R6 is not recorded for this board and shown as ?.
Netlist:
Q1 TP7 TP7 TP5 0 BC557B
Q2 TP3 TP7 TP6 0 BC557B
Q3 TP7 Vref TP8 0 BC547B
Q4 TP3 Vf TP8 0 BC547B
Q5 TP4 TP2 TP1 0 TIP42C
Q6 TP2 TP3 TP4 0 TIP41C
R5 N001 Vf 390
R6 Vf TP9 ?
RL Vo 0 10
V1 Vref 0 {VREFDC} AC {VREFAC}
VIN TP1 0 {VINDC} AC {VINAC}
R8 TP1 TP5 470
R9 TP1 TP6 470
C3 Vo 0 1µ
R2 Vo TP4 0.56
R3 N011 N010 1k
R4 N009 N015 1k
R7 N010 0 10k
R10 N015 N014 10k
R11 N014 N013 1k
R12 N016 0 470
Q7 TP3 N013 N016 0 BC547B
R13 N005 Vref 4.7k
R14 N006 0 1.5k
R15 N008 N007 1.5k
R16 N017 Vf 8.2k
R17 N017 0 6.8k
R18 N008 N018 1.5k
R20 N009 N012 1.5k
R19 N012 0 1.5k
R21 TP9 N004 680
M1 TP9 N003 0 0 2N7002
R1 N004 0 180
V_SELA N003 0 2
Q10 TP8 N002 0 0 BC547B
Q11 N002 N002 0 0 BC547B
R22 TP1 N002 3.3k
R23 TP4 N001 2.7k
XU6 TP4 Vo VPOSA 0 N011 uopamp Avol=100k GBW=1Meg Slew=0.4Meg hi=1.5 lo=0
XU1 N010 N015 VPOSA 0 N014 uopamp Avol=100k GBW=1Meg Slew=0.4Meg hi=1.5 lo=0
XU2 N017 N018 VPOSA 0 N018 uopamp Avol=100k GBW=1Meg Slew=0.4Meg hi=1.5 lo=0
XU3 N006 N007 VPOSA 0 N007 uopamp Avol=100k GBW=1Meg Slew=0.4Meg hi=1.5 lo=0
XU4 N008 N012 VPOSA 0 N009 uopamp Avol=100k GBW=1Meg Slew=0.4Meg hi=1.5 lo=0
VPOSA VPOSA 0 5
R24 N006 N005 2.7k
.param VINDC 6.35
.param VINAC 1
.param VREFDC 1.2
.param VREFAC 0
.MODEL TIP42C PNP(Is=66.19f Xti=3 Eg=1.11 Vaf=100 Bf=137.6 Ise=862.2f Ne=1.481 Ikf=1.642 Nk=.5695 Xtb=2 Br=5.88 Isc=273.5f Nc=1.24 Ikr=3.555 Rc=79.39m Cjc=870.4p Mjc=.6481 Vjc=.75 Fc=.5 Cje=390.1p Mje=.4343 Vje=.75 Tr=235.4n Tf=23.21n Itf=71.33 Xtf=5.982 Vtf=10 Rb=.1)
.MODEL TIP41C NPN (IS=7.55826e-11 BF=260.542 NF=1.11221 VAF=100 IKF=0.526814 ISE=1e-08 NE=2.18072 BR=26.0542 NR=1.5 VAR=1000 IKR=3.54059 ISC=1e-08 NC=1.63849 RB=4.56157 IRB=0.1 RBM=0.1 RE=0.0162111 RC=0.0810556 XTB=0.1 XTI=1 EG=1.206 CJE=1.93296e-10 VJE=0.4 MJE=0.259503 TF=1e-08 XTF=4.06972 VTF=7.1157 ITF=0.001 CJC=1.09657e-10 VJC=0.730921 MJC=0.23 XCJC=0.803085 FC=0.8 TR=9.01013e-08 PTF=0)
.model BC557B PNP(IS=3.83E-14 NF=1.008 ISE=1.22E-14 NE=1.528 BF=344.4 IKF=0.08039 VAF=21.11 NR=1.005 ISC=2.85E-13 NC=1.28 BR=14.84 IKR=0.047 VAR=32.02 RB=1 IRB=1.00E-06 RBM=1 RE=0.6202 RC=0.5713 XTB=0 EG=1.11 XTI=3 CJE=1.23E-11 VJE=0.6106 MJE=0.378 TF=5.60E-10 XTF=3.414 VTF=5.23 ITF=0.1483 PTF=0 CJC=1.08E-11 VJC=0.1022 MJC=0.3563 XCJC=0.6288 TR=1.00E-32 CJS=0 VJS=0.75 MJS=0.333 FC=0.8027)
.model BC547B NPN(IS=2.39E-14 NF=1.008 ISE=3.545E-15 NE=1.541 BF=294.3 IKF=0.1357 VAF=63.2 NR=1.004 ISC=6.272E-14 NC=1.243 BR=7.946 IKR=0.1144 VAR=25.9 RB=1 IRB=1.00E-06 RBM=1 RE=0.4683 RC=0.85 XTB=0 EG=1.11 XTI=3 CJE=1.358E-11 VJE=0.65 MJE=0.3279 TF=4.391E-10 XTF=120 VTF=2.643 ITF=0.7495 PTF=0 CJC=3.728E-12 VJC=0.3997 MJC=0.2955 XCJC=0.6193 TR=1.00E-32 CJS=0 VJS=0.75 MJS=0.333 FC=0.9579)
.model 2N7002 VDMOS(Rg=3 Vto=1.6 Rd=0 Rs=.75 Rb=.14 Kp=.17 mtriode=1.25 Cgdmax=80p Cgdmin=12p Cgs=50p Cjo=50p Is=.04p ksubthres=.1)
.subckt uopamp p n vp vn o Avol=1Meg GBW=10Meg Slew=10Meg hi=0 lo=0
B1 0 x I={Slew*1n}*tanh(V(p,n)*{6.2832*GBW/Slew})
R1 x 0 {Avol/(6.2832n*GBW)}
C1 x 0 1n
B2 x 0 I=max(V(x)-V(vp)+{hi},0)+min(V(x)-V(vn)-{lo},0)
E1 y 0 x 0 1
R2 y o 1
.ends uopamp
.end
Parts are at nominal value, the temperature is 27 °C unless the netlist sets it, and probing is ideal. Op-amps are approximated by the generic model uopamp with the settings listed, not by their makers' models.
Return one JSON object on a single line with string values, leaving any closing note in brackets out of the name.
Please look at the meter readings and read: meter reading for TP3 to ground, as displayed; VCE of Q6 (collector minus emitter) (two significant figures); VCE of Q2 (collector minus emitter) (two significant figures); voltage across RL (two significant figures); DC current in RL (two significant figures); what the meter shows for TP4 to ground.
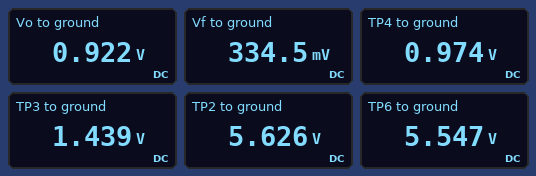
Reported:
{"meter reading for TP3 to ground, as displayed": "1.439 V", "VCE of Q6 (collector minus emitter)": "4.7 V", "VCE of Q2 (collector minus emitter)": "-4.1 V", "voltage across RL": "920 mV", "DC current in RL": "92 mA", "what the meter shows for TP4 to ground": "0.974 V"}
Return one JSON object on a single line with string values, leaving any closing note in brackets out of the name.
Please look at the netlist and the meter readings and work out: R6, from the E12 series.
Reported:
{"R6, from the E12 series": "1.8 kΩ"}
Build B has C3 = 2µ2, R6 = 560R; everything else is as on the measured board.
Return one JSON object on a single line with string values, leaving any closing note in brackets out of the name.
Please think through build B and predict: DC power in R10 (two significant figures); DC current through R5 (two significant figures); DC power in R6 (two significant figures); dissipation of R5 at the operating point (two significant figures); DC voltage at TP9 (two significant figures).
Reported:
{"DC power in R10": "860 µW", "DC current through R5": "270 µA", "DC power in R6": "37 µW", "dissipation of R5 at the operating point": "28 µW", "DC voltage at TP9": "3.2 mV"}
